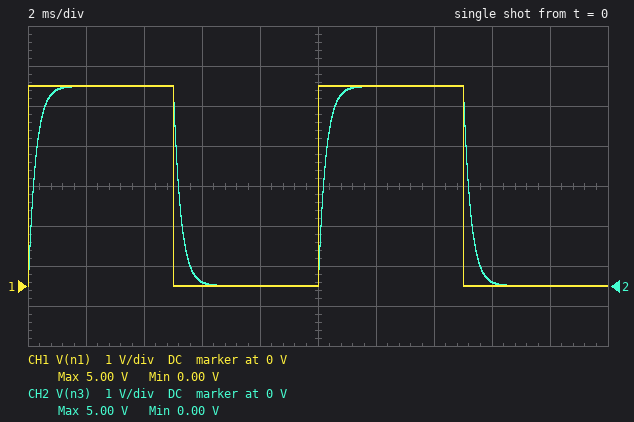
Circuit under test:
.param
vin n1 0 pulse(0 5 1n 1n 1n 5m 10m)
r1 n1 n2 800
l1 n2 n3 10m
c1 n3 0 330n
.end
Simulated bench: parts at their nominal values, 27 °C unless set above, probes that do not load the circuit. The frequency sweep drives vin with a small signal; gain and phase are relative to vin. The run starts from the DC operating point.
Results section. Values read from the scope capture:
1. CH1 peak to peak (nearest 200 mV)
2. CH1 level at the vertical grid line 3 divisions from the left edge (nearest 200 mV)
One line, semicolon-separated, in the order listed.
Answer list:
5.0 V; 0 V
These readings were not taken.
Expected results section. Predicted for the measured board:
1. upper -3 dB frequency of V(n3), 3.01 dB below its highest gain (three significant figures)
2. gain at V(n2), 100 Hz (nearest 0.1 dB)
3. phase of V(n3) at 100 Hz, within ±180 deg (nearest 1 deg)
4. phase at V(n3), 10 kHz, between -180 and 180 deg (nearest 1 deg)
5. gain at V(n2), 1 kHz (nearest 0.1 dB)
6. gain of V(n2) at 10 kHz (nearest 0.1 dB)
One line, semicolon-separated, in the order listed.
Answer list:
633 Hz; -0.1 dB; -9 deg; -126 deg; -6.7 dB; -4.6 dB
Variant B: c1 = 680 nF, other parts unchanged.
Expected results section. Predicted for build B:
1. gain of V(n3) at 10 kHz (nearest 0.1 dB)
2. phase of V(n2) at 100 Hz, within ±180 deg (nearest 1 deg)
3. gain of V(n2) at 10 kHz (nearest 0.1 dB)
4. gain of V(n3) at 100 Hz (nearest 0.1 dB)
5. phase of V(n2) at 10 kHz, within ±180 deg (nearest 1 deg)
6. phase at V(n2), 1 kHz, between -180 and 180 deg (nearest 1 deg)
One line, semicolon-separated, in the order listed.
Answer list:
-32.6 dB; -19 deg; -4.4 dB; -0.5 dB; 53 deg; -78 deg
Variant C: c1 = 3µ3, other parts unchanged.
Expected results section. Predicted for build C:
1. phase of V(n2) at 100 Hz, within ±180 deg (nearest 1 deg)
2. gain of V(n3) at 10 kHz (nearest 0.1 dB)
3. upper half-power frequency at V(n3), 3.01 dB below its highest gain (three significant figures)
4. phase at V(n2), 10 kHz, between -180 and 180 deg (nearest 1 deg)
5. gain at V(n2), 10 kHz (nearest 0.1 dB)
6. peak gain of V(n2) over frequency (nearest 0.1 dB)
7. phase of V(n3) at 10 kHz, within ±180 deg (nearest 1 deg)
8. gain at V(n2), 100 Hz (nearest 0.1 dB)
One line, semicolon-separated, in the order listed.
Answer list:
-59 deg; -46.5 dB; 60.6 Hz; 52 deg; -4.2 dB; 0 dB; -128 deg; -5.8 dB
